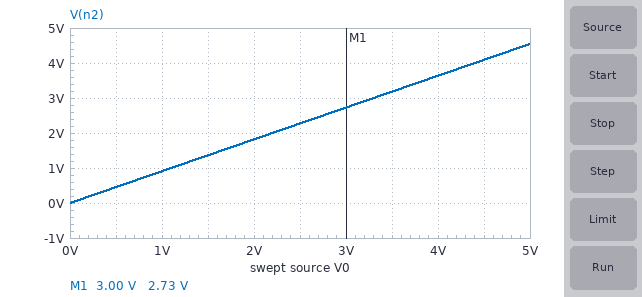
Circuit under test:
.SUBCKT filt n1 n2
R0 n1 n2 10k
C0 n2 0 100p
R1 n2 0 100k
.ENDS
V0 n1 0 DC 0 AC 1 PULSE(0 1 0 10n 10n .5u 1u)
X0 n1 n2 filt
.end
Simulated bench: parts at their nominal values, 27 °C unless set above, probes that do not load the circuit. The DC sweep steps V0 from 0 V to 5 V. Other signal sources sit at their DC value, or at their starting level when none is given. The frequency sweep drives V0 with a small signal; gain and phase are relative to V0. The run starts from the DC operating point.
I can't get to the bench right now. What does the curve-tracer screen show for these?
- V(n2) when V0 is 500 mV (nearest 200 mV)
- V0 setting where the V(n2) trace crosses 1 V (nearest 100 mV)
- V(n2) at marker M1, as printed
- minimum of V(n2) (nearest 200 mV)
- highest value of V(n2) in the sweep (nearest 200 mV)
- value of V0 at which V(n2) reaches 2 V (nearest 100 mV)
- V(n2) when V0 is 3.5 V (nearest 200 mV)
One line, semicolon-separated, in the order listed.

400 mV; 1.1 V; 2.73 V; 0 V; 4.6 V; 2.2 V; 3.2 V
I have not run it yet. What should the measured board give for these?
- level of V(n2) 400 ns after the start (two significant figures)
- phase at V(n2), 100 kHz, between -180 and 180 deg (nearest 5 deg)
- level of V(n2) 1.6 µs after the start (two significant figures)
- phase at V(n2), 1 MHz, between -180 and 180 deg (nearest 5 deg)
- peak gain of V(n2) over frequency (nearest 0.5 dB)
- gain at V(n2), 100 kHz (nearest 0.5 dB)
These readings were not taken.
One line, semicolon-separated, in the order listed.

320 mV; -30 deg; 470 mV; -80 deg; -1.0 dB; -2.0 dB
